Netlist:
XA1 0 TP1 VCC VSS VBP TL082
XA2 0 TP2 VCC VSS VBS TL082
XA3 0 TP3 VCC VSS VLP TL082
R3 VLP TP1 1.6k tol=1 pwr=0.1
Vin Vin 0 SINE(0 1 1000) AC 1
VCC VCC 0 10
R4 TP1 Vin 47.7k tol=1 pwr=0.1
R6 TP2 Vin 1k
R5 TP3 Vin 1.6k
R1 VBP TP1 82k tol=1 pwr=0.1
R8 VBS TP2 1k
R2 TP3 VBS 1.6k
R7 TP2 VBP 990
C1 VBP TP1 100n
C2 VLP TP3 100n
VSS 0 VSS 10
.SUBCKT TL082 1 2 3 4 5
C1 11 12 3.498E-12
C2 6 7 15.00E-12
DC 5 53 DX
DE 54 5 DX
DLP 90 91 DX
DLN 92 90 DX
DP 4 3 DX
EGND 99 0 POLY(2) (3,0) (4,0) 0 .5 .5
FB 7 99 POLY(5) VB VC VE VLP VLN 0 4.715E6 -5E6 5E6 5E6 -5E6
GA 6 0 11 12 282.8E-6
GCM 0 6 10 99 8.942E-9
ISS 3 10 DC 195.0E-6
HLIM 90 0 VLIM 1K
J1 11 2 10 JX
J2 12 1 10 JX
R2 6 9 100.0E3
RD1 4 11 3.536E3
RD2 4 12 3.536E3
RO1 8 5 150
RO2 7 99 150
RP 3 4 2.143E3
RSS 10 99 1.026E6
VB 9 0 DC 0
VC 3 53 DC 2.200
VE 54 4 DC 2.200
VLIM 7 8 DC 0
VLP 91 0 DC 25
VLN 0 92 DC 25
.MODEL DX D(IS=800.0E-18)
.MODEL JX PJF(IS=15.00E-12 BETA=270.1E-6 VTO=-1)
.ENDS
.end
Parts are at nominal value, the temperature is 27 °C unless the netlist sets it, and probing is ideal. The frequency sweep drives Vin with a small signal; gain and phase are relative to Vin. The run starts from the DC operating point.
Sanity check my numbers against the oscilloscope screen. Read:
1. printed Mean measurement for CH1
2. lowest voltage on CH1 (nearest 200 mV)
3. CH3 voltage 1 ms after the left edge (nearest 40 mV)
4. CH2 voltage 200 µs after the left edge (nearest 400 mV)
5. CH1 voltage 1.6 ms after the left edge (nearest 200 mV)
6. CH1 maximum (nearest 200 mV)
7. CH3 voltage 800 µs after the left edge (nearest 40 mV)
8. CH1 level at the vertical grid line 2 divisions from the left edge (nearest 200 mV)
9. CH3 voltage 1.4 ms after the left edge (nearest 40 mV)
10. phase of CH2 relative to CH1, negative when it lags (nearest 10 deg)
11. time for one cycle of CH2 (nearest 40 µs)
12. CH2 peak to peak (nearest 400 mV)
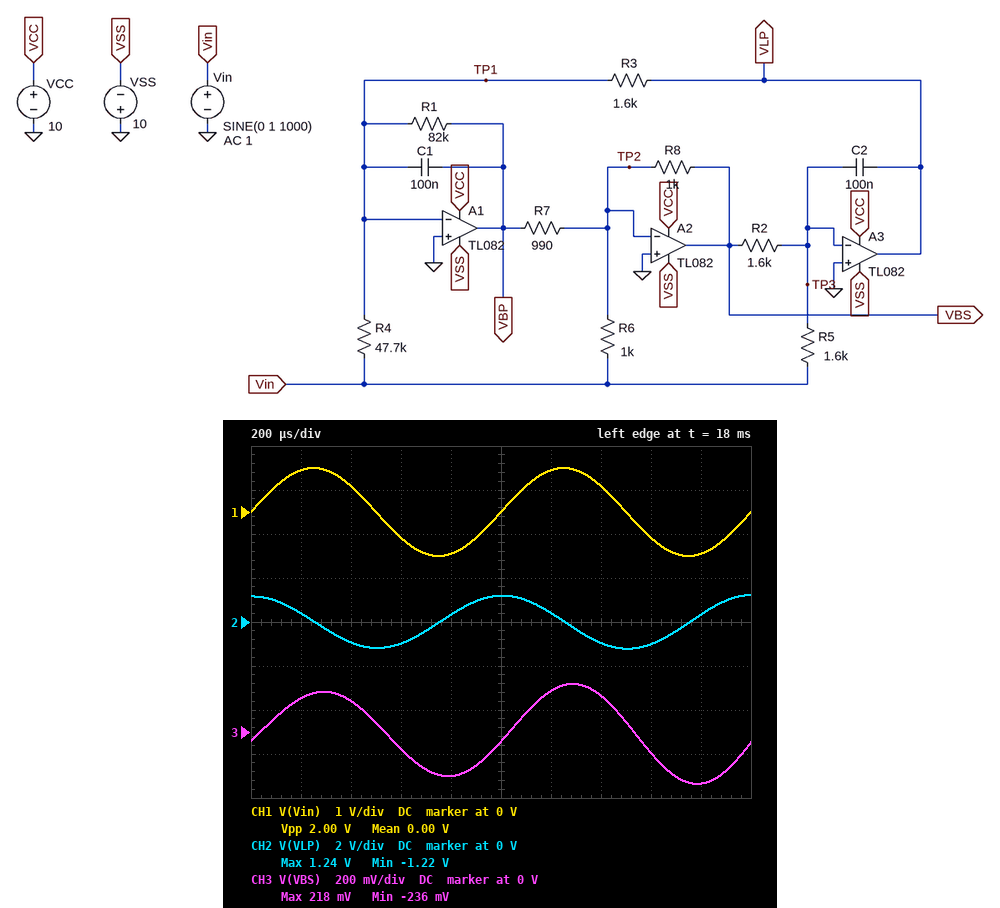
0.00 V
-1.0 V
-40 mV
400 mV
-600 mV
1.0 V
-200 mV
600 mV
160 mV
90 deg
1.00 ms
2.4 V
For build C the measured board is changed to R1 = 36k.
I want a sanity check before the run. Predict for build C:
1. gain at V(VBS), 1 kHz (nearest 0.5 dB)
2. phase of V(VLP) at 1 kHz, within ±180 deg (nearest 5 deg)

-12.5 dB
90 deg
